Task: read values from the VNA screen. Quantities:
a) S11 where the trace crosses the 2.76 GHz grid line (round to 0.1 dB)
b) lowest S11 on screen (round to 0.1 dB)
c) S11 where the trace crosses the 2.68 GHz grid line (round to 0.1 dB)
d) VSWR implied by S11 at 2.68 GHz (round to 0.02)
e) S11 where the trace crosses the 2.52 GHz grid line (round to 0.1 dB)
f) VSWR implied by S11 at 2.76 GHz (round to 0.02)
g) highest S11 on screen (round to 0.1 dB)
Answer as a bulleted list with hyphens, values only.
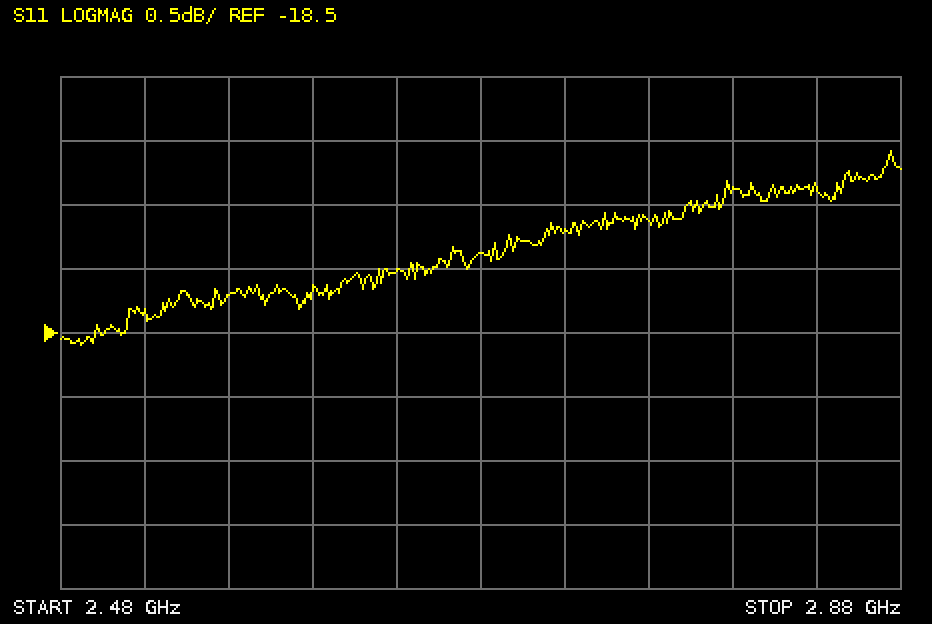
- -17.6 dB
- -18.6 dB
- -17.9 dB
- 1.30
- -18.3 dB
- 1.30
- -17.1 dB
